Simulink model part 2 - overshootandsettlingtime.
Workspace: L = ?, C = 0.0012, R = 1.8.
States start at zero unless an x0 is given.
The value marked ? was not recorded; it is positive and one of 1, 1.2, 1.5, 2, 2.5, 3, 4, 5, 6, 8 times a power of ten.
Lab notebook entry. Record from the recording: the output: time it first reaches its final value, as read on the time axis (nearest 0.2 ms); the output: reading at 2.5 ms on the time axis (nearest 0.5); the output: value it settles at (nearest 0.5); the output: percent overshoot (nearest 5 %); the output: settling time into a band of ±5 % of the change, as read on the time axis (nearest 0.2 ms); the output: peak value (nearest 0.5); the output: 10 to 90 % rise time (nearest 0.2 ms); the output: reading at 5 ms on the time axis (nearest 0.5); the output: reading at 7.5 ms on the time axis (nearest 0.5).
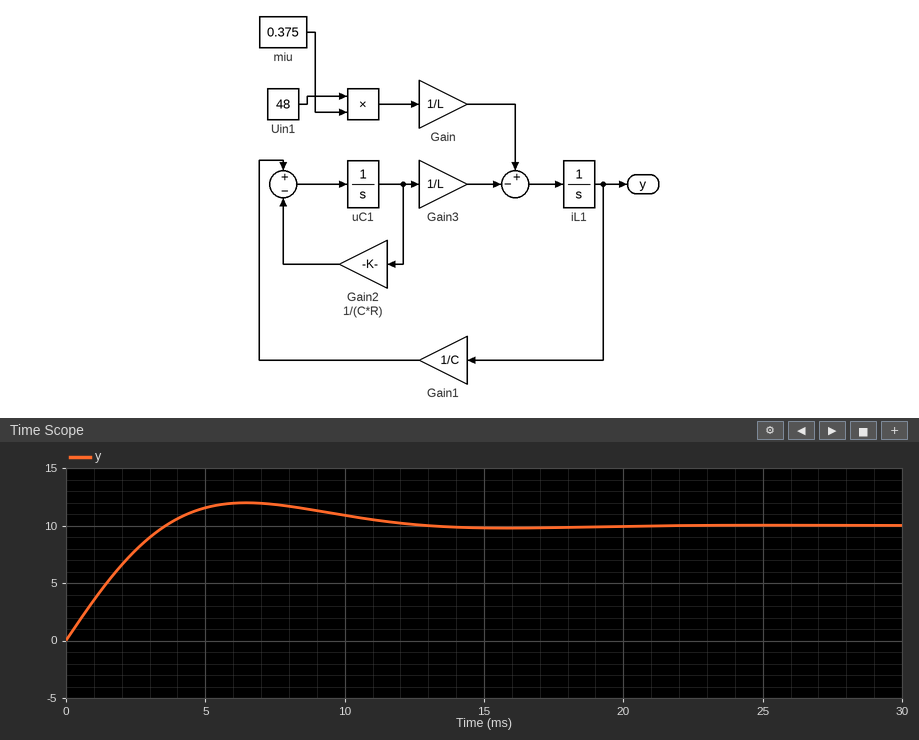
3.6 ms
8.0
10.0
20 %
11.0 ms
12.0
2.8 ms
11.5
12.0
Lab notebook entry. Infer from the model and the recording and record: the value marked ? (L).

0.005
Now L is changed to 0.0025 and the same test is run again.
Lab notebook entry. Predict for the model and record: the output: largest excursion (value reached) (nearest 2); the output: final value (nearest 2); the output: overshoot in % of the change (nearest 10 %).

16
10
50 %
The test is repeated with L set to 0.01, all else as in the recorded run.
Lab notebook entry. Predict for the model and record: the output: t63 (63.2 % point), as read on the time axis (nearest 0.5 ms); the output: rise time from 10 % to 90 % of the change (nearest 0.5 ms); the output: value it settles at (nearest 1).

4.0 ms
7.0 ms
10
